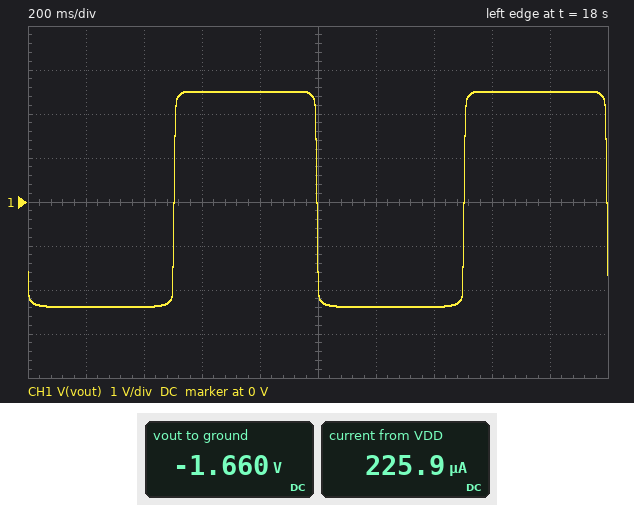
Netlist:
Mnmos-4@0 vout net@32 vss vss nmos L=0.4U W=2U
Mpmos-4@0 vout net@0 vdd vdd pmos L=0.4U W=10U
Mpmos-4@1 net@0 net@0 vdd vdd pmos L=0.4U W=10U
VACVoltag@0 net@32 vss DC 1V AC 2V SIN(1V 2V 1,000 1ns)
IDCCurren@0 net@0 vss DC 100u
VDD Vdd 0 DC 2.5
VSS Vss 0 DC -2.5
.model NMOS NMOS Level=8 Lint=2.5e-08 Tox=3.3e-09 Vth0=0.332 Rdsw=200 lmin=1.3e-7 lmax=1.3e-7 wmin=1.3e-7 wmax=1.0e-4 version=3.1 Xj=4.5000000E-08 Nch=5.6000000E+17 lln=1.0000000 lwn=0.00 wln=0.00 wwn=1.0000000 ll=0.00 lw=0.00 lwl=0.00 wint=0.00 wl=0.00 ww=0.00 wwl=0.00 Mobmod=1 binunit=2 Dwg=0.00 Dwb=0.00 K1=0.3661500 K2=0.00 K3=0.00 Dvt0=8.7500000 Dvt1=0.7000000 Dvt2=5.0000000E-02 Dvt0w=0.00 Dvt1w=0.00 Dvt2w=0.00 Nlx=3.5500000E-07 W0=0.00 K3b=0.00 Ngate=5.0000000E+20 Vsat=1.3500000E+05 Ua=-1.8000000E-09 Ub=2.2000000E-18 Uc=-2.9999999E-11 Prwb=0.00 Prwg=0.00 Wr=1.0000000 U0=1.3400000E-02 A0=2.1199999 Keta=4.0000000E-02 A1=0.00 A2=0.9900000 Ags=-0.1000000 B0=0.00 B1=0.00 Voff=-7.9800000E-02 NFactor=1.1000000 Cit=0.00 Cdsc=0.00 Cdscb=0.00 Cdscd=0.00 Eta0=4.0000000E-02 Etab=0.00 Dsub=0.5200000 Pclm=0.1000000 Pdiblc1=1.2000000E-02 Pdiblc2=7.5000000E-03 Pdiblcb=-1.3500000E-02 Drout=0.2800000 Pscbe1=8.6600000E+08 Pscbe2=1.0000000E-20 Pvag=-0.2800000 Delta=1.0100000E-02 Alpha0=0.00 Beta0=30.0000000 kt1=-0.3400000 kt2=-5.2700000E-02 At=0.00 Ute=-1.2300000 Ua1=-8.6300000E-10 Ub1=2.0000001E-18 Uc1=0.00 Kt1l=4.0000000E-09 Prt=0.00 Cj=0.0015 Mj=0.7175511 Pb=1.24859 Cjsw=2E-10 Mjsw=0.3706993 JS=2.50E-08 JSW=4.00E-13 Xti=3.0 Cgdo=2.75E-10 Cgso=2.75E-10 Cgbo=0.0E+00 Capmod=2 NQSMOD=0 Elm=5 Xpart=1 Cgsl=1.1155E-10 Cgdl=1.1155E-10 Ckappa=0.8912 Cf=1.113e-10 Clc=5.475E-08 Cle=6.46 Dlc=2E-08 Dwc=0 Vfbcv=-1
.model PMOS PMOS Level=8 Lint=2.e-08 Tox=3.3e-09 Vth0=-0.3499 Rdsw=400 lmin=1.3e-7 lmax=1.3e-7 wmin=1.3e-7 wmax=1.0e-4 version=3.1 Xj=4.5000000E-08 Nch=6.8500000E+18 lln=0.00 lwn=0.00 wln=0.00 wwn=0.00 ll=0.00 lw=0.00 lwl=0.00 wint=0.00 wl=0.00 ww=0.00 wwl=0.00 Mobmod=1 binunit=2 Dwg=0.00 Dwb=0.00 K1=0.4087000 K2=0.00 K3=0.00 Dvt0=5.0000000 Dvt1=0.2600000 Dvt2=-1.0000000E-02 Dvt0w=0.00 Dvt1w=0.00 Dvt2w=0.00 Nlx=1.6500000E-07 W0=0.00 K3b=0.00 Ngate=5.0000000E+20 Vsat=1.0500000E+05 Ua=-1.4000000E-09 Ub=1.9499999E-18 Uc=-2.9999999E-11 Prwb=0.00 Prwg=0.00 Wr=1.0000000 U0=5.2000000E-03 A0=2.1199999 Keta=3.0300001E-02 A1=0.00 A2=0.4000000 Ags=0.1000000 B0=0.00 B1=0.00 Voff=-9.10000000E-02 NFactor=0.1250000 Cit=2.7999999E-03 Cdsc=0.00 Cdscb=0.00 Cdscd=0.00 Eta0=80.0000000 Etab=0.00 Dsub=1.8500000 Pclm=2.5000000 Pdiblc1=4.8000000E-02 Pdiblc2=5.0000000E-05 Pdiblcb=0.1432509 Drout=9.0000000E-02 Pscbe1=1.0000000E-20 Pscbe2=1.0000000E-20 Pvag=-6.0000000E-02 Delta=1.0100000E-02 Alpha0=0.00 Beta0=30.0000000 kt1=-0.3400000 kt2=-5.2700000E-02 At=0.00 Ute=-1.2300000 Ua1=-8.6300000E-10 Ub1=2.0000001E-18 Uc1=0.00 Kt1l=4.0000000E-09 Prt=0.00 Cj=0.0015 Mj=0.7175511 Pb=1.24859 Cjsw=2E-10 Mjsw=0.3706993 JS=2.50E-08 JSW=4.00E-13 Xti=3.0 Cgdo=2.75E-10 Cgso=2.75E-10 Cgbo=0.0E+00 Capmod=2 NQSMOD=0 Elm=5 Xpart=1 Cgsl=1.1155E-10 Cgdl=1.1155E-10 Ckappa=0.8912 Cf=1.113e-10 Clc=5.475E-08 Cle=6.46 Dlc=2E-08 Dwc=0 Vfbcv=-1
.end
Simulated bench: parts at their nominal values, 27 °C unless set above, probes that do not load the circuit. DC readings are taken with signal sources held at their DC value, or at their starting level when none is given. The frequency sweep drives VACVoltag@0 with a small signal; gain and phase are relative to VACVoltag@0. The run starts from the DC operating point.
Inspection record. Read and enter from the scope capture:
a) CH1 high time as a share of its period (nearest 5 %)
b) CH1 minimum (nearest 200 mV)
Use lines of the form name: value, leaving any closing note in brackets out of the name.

CH1 high time as a share of its period: 50 %
CH1 minimum: -2.4 V
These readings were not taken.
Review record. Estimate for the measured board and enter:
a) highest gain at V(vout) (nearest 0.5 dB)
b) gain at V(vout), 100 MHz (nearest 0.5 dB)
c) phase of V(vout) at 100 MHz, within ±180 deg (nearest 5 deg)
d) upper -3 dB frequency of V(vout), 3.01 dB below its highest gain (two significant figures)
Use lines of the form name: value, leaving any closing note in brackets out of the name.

highest gain at V(vout): 31.0 dB
gain at V(vout), 100 MHz: 30.0 dB
phase of V(vout) at 100 MHz, within ±180 deg: 150 deg
upper -3 dB frequency of V(vout), 3.01 dB below its highest gain: 170 MHz
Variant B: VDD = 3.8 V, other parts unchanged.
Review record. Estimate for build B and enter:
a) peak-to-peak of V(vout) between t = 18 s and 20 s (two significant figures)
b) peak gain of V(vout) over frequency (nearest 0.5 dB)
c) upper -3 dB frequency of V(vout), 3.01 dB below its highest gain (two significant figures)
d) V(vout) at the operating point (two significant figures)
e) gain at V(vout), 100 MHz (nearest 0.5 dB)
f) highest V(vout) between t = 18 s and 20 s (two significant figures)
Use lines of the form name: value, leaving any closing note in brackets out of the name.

peak-to-peak of V(vout) between t = 18 s and 20 s: 6.2 V
peak gain of V(vout) over frequency: 32.0 dB
upper -3 dB frequency of V(vout), 3.01 dB below its highest gain: 160 MHz
V(vout) at the operating point: -830 mV
gain at V(vout), 100 MHz: 30.5 dB
highest V(vout) between t = 18 s and 20 s: 3.8 V
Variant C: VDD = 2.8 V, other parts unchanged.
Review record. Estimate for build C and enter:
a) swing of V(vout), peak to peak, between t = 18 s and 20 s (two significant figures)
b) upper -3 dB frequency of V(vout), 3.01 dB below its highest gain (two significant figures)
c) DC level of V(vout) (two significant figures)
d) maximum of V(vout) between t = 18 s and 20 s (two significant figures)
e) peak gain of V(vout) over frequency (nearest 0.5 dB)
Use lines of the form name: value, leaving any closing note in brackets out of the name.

swing of V(vout), peak to peak, between t = 18 s and 20 s: 5.2 V
upper -3 dB frequency of V(vout), 3.01 dB below its highest gain: 160 MHz
DC level of V(vout): -1.5 V
maximum of V(vout) between t = 18 s and 20 s: 2.8 V
peak gain of V(vout) over frequency: 31.5 dB
